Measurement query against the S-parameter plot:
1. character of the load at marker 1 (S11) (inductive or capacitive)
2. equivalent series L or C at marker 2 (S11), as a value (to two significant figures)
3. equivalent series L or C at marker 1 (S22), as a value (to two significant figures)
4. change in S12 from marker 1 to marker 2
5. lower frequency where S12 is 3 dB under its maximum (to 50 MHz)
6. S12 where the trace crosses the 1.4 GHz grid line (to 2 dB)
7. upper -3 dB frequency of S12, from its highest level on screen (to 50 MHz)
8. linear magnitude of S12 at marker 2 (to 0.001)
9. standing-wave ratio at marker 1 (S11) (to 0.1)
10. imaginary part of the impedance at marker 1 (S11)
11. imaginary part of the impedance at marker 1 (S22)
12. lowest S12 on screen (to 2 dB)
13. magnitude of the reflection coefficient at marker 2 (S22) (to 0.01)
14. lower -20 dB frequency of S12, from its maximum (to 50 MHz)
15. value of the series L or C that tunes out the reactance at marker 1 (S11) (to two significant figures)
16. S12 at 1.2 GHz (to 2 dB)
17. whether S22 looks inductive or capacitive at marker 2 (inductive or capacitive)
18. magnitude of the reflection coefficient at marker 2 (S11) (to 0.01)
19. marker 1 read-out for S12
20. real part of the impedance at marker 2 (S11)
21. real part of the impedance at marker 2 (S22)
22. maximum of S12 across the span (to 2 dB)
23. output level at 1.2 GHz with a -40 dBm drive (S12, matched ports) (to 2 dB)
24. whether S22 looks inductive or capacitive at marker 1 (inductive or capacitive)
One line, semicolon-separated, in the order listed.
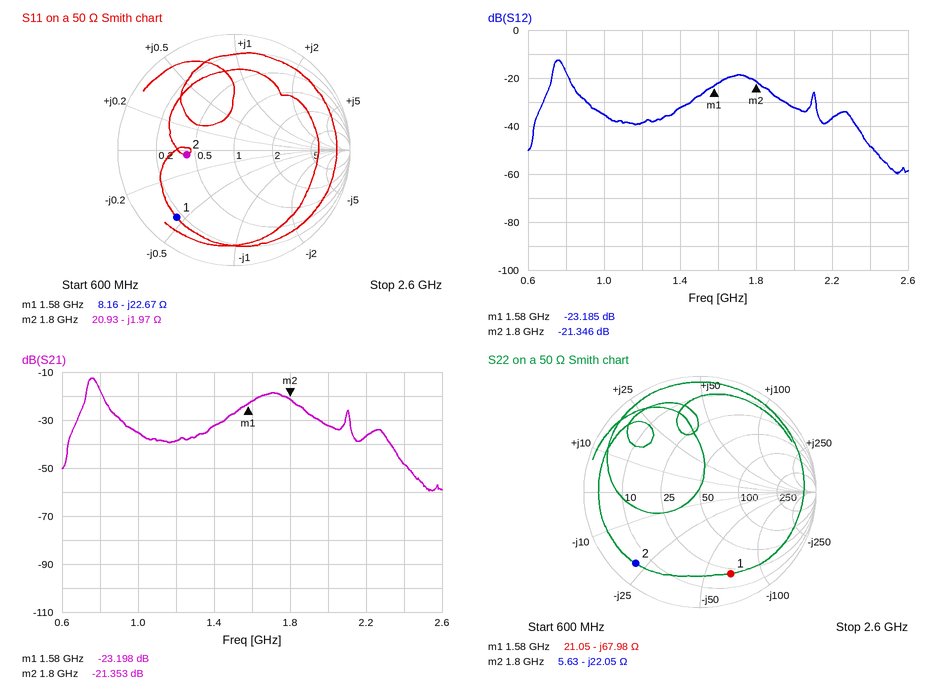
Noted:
capacitive; 45 pF; 1.5 pF; 1.839 dB; 750 MHz; -32 dB; 800 MHz; 0.086; 7.4; -22.67 Ω; -67.98 Ω; -60 dB; 0.83; 650 MHz; 2.3 nH; -38 dB; capacitive; 0.41; -23.185 dB; 20.93 Ω; 5.63 Ω; -12 dB; -78 dBm; capacitive
